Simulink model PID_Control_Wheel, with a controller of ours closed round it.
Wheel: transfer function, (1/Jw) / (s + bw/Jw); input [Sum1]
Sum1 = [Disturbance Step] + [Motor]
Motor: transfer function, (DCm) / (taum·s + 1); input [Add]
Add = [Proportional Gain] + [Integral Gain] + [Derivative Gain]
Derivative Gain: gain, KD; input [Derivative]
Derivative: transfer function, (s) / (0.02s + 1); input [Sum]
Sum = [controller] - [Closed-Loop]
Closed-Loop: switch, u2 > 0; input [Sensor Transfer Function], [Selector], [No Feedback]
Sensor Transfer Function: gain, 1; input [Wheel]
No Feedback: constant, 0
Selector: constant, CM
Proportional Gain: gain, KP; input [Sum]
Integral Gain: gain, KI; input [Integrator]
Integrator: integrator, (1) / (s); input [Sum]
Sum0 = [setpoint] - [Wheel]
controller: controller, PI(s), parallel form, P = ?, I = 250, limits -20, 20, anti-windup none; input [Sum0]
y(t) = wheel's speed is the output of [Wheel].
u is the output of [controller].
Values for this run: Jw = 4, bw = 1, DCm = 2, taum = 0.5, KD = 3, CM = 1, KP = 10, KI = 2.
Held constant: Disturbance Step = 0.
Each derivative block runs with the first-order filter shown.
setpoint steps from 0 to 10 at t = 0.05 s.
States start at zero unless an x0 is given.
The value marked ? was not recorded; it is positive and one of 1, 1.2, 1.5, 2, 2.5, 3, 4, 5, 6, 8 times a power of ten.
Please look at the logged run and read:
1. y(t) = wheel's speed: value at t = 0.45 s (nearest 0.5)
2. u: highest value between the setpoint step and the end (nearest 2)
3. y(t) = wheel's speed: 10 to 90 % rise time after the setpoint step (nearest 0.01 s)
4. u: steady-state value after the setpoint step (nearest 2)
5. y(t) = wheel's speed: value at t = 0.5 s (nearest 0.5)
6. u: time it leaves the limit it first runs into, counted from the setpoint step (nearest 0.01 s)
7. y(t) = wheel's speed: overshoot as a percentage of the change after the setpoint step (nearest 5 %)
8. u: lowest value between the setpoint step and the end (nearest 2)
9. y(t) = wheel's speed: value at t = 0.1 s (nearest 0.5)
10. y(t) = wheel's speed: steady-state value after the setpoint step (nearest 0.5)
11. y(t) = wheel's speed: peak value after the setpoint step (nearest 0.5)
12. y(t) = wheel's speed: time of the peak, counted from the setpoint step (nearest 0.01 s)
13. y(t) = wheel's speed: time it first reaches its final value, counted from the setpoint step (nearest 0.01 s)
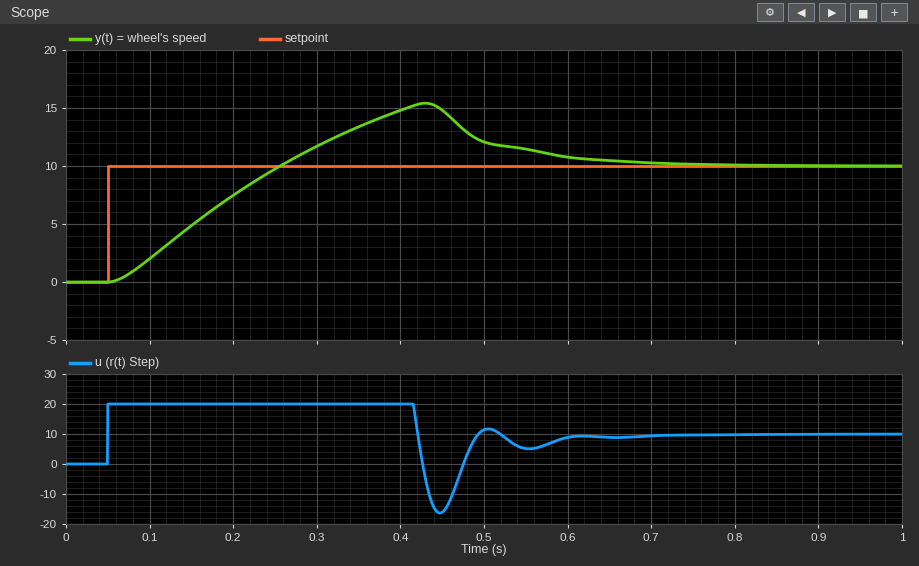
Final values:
15.0
20
0.15 s
10
12.0
0.37 s
55 %
-16
2.0
10.0
15.5
0.38 s
0.21 s
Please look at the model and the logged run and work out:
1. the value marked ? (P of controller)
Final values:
25
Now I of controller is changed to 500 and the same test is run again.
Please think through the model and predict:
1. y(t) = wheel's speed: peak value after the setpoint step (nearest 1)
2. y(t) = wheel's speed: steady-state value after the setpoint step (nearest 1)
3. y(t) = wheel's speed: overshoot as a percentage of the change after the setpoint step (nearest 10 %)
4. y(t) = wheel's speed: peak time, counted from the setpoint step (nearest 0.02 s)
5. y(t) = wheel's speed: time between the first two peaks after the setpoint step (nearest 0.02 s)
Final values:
16
10
60 %
0.42 s
0.20 s
